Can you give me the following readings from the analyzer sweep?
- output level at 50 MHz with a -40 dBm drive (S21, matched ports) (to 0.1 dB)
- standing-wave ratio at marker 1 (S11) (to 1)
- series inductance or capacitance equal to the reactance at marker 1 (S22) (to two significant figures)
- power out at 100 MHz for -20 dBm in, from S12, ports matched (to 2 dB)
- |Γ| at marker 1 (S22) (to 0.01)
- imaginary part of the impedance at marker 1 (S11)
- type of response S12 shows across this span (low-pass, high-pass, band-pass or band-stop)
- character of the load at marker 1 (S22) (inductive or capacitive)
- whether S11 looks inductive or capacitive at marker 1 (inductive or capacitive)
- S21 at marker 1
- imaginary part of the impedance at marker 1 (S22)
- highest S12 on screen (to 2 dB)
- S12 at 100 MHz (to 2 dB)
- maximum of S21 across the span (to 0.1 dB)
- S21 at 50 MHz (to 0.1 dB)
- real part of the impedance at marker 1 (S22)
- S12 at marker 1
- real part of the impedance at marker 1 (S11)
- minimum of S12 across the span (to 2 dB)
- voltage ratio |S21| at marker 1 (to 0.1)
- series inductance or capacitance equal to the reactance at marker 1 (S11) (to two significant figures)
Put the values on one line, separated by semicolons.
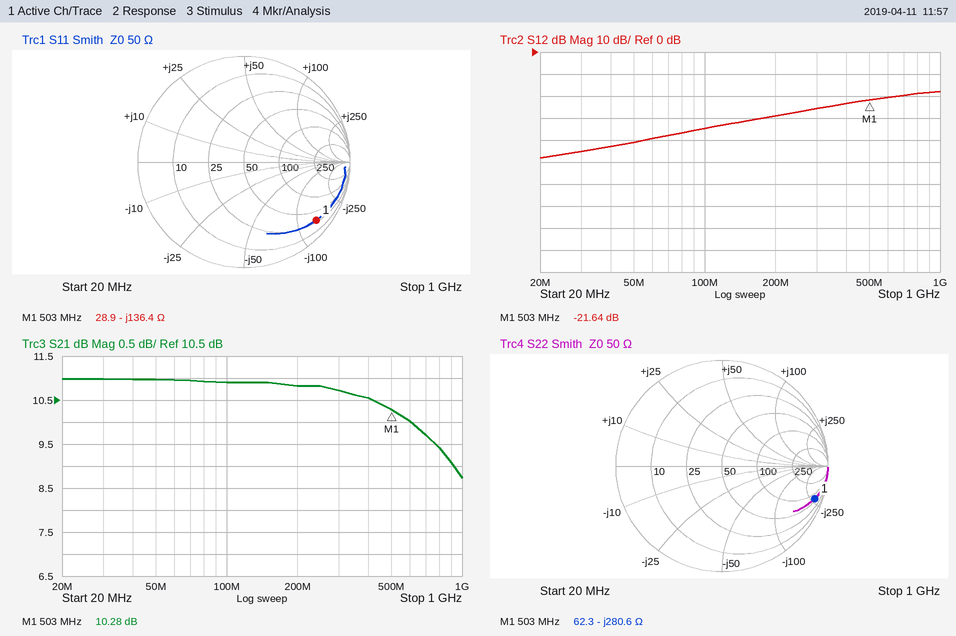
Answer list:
-29.0 dBm; 15; 1.1 pF; -54 dBm; 0.93; -136.4 Ω; high-pass; capacitive; capacitive; 10.28 dB; -280.6 Ω; -18 dB; -34 dB; 11.0 dB; 11.0 dB; 62.3 Ω; -21.64 dB; 28.9 Ω; -48 dB; 3.3; 2.3 pF
